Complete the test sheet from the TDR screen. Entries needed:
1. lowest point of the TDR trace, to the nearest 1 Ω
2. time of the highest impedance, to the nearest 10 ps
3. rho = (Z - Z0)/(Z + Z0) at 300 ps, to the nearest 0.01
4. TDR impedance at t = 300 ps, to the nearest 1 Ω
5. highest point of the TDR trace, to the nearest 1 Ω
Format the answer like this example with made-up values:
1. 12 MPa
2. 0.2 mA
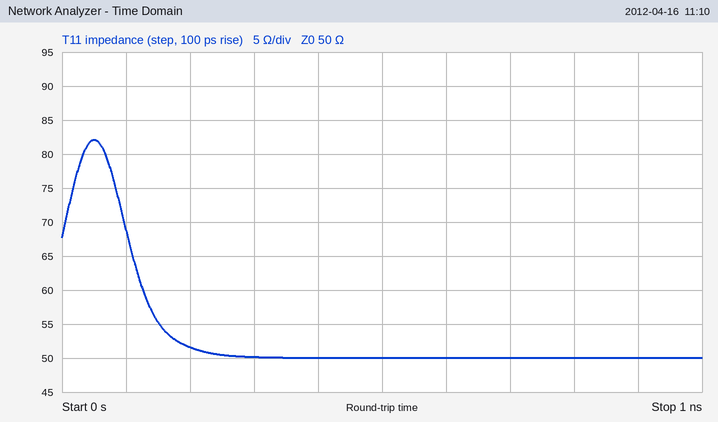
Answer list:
1. 50 Ω
2. 50 ps
3. 0.00
4. 50 Ω
5. 82 Ω
